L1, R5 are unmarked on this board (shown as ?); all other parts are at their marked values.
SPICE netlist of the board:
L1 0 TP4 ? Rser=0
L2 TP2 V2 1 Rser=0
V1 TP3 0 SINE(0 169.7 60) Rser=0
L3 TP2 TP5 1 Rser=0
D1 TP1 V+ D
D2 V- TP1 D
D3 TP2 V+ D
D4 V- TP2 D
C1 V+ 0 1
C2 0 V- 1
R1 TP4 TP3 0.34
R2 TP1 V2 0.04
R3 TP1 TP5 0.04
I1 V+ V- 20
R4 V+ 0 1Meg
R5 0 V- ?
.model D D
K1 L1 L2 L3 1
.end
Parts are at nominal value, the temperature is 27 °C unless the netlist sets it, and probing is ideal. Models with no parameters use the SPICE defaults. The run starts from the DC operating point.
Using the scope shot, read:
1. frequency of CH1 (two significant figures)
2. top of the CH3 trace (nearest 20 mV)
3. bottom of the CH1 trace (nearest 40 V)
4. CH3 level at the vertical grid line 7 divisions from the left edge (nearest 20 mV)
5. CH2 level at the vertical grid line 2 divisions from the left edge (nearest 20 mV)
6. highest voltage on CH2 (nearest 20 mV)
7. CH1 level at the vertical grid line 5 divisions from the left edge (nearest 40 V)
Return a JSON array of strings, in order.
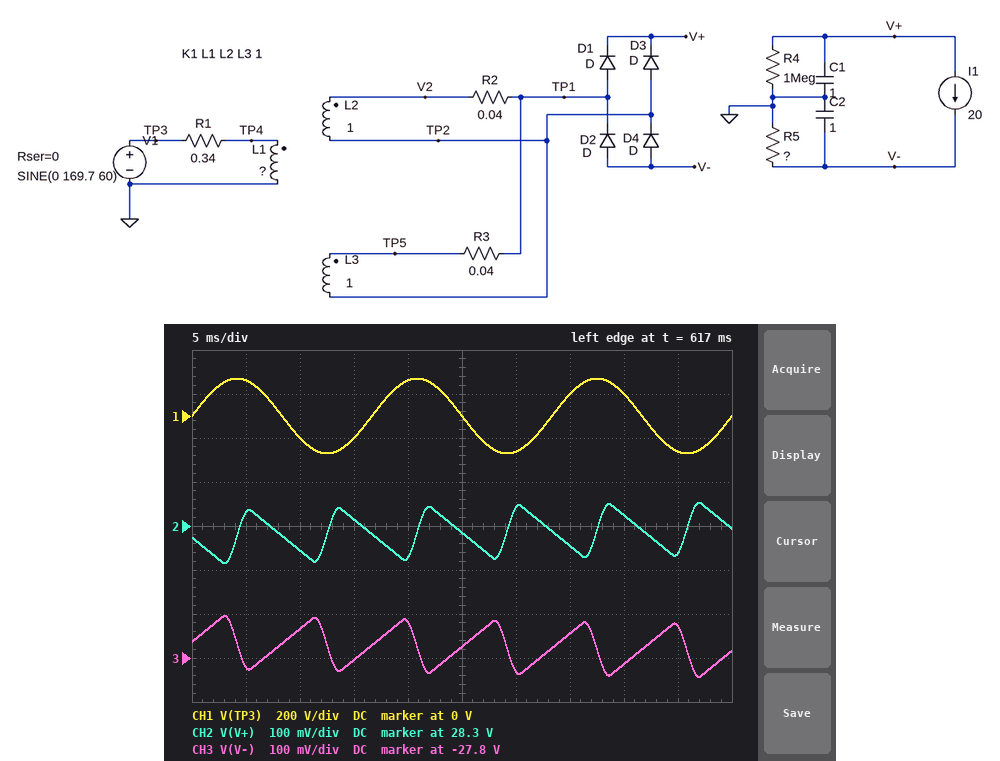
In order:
["60 Hz", "-27.70 V", "-160 V", "-27.74 V", "28.24 V", "28.36 V", "0 V"]
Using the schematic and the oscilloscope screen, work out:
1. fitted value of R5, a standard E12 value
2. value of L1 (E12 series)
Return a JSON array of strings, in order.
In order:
["1.8 MΩ", "6.8 H"]
